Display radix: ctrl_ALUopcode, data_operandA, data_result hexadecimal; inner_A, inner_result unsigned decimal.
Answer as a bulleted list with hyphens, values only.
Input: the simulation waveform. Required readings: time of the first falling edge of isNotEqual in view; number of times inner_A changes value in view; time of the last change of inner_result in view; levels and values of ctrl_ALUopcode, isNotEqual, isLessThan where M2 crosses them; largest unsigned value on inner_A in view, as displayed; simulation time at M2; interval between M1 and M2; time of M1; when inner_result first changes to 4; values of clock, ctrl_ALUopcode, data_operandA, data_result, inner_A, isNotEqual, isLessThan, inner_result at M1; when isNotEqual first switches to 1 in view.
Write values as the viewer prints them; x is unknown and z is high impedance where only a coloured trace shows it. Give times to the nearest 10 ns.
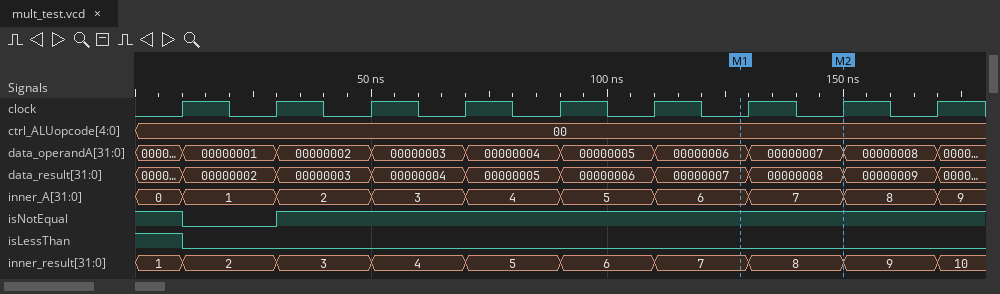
- 10 ns
- 9
- 170 ns
- ctrl_ALUopcode=00, isNotEqual=1, isLessThan=0
- 9
- 150 ns
- 20 ns
- 130 ns
- 50 ns
- clock=0, ctrl_ALUopcode=00, data_operandA=00000006, data_result=00000007, inner_A=6, isNotEqual=1, isLessThan=0, inner_result=7
- 30 ns
